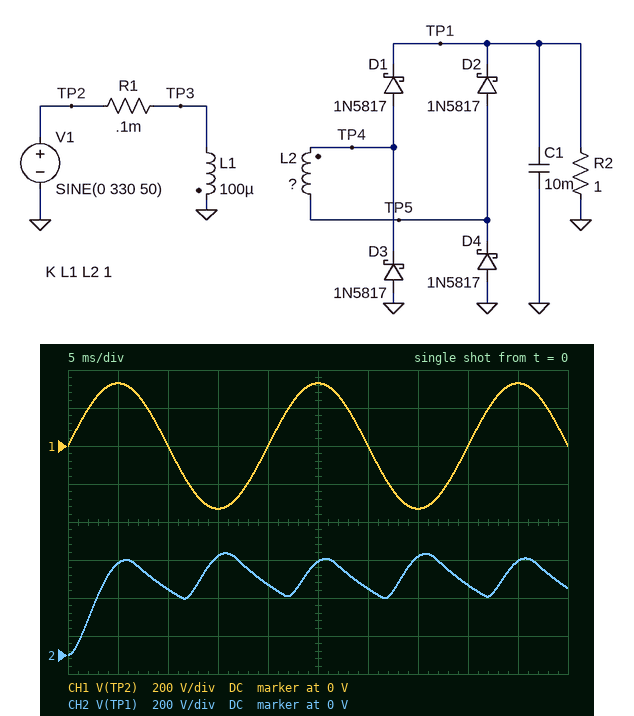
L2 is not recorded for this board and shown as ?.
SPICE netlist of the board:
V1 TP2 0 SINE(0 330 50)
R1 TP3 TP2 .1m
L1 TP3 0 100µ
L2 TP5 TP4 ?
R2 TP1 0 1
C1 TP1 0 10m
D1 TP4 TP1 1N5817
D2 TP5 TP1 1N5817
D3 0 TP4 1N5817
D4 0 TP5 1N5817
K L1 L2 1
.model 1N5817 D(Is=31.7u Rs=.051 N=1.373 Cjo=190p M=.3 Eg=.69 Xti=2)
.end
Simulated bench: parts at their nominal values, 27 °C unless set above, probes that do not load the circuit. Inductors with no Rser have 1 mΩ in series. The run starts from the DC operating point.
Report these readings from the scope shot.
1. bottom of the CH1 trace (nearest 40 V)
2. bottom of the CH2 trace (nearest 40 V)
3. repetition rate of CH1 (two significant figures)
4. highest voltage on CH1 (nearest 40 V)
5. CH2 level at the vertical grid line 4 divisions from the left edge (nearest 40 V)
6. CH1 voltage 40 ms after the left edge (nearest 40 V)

-320 V
0 V
50 Hz
320 V
360 V
0 V
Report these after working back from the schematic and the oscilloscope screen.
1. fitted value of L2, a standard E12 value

330 µH
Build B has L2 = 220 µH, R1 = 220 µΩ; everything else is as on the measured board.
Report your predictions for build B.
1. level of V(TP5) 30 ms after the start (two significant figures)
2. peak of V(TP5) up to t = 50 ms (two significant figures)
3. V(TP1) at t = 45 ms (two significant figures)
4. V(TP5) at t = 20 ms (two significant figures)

130 V
440 V
400 V
150 V
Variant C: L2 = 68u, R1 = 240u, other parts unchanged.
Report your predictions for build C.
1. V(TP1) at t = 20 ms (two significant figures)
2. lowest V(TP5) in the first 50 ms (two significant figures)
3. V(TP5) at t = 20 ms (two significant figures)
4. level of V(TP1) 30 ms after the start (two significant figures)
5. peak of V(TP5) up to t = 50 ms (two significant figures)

170 V
-31 V
85 V
160 V
250 V
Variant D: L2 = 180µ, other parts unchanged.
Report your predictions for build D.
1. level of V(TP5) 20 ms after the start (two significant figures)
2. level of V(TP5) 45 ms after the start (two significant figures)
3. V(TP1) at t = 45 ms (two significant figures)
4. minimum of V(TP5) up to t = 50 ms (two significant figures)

140 V
400 V
370 V
-49 V
